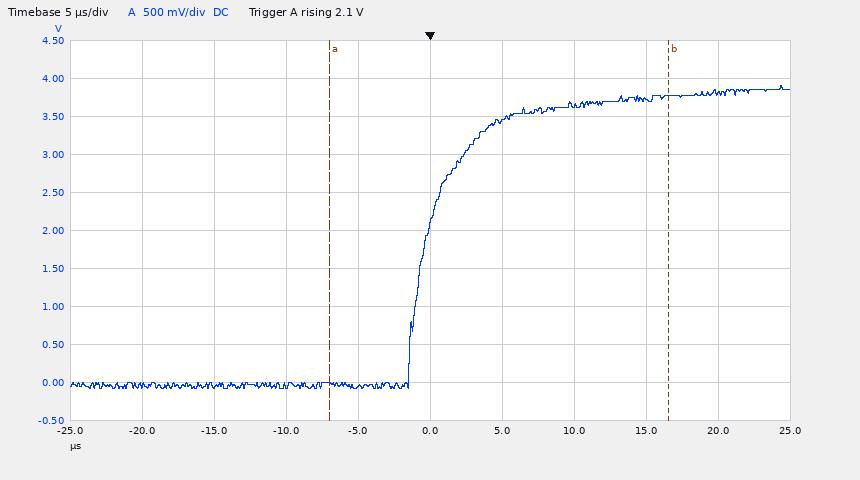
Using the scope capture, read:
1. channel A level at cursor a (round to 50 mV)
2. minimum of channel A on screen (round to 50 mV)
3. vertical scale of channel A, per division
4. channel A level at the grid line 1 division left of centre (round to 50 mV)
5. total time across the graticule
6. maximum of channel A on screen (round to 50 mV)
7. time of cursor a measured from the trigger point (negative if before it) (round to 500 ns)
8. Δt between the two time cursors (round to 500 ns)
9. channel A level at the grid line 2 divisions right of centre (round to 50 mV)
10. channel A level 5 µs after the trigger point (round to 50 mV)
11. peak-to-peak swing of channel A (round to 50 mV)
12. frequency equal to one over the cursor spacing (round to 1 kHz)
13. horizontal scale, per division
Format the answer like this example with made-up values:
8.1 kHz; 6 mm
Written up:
0 mV; -100 mV; 500 mV; -50 mV; 50 µs; 3.90 V; -7.0 µs; 23.5 µs; 3.65 V; 3.45 V; 4.00 V; 43 kHz; 5 µs
